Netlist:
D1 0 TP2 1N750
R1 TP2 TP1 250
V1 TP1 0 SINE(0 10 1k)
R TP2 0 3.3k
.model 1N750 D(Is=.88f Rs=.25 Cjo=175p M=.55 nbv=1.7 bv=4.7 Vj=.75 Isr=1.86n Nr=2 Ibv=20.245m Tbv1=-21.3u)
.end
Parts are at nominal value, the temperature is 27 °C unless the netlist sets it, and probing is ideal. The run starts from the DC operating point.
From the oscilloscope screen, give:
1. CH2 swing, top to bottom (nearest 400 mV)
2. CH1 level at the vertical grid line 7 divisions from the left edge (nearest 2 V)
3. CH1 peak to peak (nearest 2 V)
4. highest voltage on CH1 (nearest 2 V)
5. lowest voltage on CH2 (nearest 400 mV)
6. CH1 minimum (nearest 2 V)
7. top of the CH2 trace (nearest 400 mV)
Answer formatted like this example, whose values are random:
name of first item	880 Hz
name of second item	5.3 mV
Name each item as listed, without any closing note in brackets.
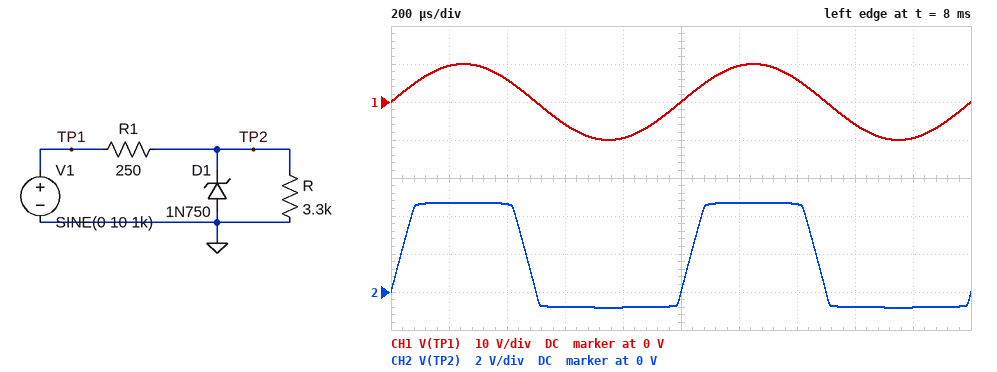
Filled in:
CH2 swing, top to bottom	5.6 V
CH1 level at the vertical grid line 7 divisions from the left edge	6 V
CH1 peak to peak	20 V
highest voltage on CH1	10 V
lowest voltage on CH2	-800 mV
CH1 minimum	-10 V
top of the CH2 trace	4.8 V
